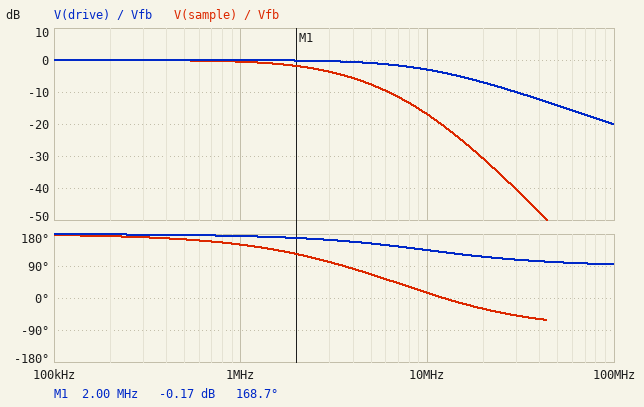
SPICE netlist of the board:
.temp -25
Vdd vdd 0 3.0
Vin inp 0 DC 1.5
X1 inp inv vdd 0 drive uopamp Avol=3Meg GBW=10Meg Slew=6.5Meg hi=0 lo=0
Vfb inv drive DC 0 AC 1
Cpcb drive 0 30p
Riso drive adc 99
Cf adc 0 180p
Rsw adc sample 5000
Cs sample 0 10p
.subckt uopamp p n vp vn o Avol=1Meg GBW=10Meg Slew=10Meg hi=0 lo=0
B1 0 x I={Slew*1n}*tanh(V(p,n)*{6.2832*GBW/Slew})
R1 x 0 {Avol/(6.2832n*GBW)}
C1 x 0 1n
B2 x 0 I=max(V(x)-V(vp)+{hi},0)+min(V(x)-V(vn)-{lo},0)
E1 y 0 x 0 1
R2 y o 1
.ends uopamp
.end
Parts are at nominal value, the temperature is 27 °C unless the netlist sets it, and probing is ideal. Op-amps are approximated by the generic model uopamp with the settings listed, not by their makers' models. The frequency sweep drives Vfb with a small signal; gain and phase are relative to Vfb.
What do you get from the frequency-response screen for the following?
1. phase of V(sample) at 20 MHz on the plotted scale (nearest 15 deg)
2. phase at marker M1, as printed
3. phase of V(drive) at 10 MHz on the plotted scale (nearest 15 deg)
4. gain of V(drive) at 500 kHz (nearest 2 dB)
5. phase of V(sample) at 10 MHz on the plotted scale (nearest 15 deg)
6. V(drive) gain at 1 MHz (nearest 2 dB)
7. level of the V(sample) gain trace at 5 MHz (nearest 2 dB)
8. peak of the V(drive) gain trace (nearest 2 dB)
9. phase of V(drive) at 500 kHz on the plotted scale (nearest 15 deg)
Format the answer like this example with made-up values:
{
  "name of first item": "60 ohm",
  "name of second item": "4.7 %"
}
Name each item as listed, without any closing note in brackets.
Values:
{
  "phase of V(sample) at 20 MHz on the plotted scale": "-30 deg",
  "phase at marker M1, as printed": "168.7 deg",
  "phase of V(drive) at 10 MHz on the plotted scale": "135 deg",
  "gain of V(drive) at 500 kHz": "0 dB",
  "phase of V(sample) at 10 MHz on the plotted scale": "15 deg",
  "V(drive) gain at 1 MHz": "0 dB",
  "level of the V(sample) gain trace at 5 MHz": "-8 dB",
  "peak of the V(drive) gain trace": "0 dB",
  "phase of V(drive) at 500 kHz on the plotted scale": "180 deg"
}
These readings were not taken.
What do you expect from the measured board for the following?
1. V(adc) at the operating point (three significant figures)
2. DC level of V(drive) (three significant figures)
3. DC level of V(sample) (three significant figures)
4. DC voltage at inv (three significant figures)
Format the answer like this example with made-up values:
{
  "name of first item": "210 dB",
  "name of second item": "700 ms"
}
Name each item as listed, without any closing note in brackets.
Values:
{
  "V(adc) at the operating point": "1.50 V",
  "DC level of V(drive)": "1.50 V",
  "DC level of V(sample)": "1.50 V",
  "DC voltage at inv": "1.50 V"
}
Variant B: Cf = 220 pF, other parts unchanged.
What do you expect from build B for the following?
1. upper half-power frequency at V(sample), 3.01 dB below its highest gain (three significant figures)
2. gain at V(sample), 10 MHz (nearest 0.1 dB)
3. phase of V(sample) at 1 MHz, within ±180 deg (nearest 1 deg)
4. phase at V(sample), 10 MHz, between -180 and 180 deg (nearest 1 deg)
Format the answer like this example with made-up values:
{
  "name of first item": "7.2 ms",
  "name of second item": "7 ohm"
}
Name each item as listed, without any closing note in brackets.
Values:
{
  "upper half-power frequency at V(sample), 3.01 dB below its highest gain": "2.55 MHz",
  "gain at V(sample), 10 MHz": "-18.0 dB",
  "phase of V(sample) at 1 MHz, within ±180 deg": "149 deg",
  "phase at V(sample), 10 MHz, between -180 and 180 deg": "9 deg"
}
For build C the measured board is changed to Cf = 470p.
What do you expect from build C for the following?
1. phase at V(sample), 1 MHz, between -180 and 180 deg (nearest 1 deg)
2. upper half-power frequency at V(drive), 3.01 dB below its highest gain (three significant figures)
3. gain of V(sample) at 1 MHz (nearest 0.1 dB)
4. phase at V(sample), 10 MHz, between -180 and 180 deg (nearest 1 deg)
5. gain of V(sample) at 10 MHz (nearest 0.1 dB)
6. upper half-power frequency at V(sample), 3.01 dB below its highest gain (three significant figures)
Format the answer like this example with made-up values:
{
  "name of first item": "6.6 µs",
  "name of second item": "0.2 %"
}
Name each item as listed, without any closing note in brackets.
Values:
{
  "phase at V(sample), 1 MHz, between -180 and 180 deg": "140 deg",
  "upper half-power frequency at V(drive), 3.01 dB below its highest gain": "9.96 MHz",
  "gain of V(sample) at 1 MHz": "-0.8 dB",
  "phase at V(sample), 10 MHz, between -180 and 180 deg": "-9 deg",
  "gain of V(sample) at 10 MHz": "-23.2 dB",
  "upper half-power frequency at V(sample), 3.01 dB below its highest gain": "2.02 MHz"
}
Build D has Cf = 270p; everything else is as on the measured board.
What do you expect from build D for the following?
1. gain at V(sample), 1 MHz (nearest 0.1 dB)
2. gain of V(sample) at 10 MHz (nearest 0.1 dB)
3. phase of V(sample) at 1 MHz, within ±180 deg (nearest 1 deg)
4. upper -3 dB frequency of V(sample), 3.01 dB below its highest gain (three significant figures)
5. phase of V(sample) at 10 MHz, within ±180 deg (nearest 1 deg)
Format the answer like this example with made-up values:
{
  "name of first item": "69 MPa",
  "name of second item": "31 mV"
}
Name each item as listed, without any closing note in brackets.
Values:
{
  "gain at V(sample), 1 MHz": "-0.6 dB",
  "gain of V(sample) at 10 MHz": "-19.3 dB",
  "phase of V(sample) at 1 MHz, within ±180 deg": "147 deg",
  "upper -3 dB frequency of V(sample), 3.01 dB below its highest gain": "2.44 MHz",
  "phase of V(sample) at 10 MHz, within ±180 deg": "3 deg"
}
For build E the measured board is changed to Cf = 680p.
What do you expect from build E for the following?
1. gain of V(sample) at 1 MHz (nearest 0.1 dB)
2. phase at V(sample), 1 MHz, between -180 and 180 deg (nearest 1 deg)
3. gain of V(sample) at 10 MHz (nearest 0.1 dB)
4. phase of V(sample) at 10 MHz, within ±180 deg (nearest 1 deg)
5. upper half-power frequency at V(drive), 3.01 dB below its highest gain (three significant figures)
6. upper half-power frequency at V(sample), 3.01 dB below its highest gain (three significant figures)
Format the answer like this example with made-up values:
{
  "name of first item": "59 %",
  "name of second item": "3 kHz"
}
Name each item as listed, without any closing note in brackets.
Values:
{
  "gain of V(sample) at 1 MHz": "-1.2 dB",
  "phase at V(sample), 1 MHz, between -180 and 180 deg": "134 deg",
  "gain of V(sample) at 10 MHz": "-26.2 dB",
  "phase of V(sample) at 10 MHz, within ±180 deg": "-14 deg",
  "upper half-power frequency at V(drive), 3.01 dB below its highest gain": "9.95 MHz",
  "upper half-power frequency at V(sample), 3.01 dB below its highest gain": "1.68 MHz"
}
